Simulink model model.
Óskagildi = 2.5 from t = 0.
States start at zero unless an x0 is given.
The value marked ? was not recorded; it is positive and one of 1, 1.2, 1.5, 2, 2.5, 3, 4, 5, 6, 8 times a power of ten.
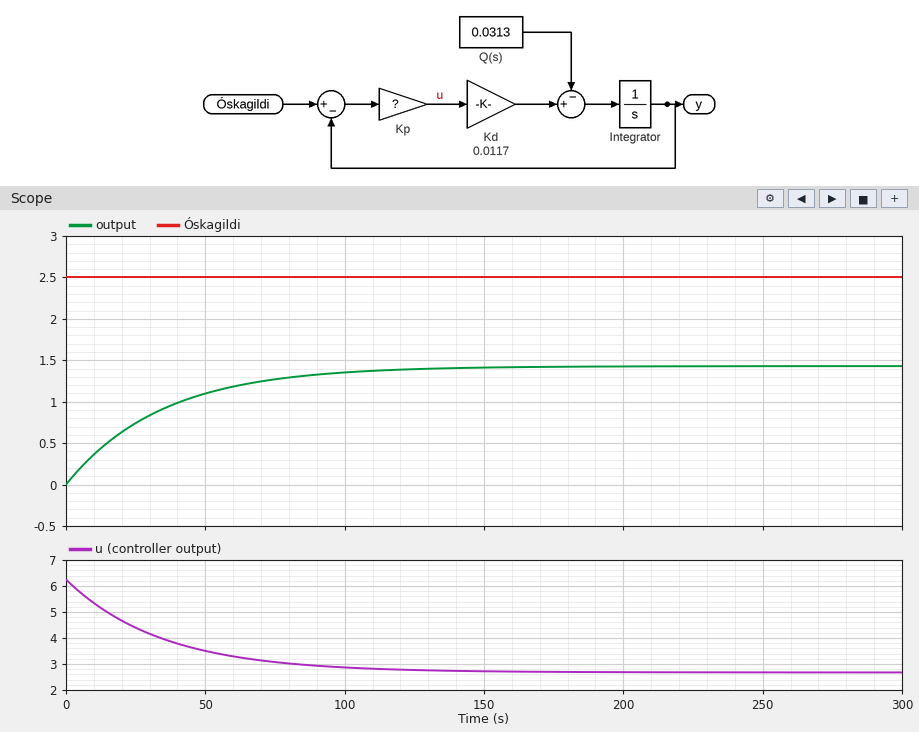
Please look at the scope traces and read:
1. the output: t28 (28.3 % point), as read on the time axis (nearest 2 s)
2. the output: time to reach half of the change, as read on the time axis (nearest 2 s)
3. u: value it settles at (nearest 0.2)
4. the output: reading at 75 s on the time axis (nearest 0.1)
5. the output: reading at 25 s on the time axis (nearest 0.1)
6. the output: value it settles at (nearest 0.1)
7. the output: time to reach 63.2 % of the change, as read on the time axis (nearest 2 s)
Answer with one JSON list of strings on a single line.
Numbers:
["12 s", "24 s", "2.6", "1.3", "0.7", "1.4", "34 s"]
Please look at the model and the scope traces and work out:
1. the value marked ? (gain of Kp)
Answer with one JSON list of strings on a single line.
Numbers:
["2.5"]
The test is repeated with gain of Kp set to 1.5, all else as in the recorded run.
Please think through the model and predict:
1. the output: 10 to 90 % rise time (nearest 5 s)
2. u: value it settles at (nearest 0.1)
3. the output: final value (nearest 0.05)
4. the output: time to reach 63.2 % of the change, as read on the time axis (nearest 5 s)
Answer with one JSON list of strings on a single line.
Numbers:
["125 s", "2.7", "0.70", "55 s"]
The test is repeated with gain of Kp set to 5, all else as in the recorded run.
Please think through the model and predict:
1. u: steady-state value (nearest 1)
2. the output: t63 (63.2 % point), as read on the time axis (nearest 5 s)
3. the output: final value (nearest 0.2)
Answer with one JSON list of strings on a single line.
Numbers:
["3", "15 s", "2.0"]
